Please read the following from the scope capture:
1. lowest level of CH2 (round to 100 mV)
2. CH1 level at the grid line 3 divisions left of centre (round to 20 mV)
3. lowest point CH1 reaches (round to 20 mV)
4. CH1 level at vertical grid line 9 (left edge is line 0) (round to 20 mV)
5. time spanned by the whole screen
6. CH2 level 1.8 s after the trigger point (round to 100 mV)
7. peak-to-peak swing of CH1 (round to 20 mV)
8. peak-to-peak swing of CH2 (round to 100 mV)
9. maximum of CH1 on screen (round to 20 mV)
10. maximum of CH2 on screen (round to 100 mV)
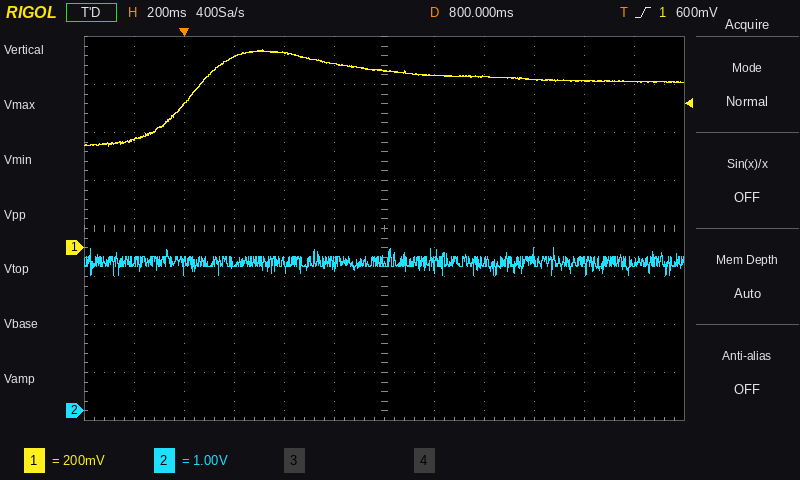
2.8 V
800 mV
420 mV
700 mV
2.4 s
3.1 V
400 mV
600 mV
820 mV
3.4 V
